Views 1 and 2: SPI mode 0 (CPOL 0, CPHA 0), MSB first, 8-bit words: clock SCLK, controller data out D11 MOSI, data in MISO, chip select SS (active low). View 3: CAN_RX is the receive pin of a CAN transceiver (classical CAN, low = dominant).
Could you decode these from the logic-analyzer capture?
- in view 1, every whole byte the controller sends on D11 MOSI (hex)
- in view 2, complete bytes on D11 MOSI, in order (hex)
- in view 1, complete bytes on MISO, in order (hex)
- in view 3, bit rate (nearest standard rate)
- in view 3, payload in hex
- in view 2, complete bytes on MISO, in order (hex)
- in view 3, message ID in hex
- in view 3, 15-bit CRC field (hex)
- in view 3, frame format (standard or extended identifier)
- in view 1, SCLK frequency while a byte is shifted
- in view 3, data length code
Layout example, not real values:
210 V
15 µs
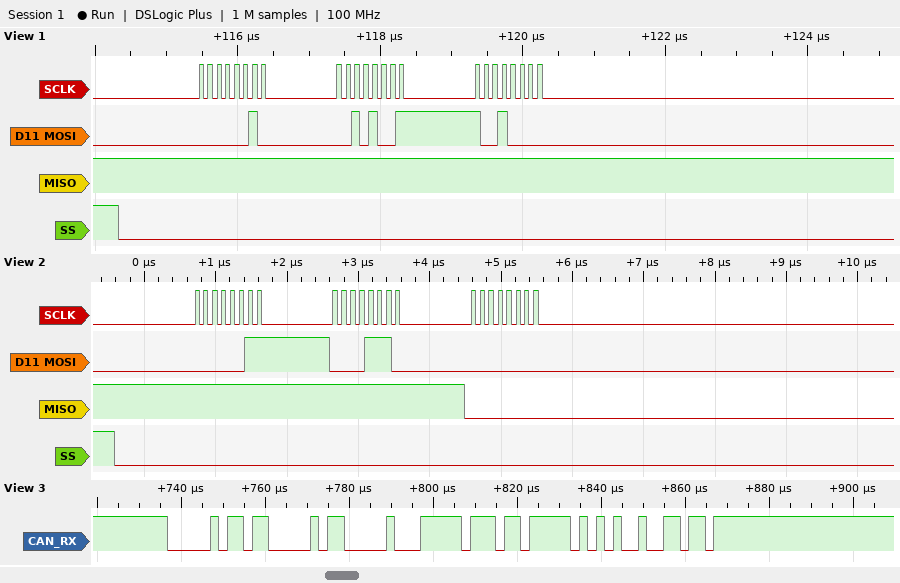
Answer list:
0x02 0x29 0x90
0x03 0x0E 0x00
0xFF 0xFF 0xFF
500 kbit/s
00 FF 6F
0xFF 0xFF 0x00
0x036
0x6A4D
standard
8 MHz
3
